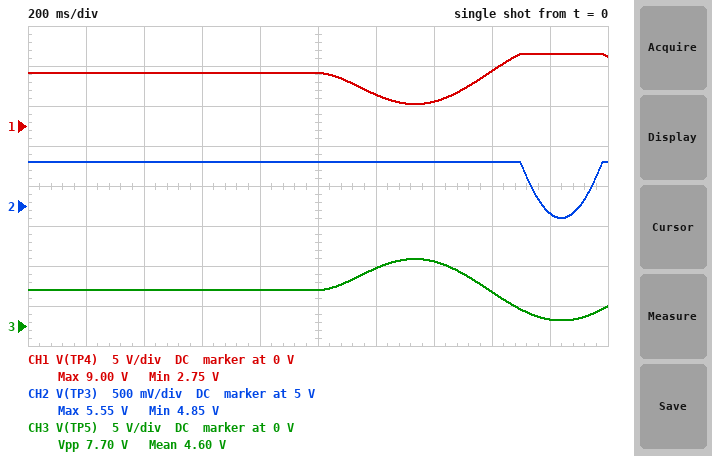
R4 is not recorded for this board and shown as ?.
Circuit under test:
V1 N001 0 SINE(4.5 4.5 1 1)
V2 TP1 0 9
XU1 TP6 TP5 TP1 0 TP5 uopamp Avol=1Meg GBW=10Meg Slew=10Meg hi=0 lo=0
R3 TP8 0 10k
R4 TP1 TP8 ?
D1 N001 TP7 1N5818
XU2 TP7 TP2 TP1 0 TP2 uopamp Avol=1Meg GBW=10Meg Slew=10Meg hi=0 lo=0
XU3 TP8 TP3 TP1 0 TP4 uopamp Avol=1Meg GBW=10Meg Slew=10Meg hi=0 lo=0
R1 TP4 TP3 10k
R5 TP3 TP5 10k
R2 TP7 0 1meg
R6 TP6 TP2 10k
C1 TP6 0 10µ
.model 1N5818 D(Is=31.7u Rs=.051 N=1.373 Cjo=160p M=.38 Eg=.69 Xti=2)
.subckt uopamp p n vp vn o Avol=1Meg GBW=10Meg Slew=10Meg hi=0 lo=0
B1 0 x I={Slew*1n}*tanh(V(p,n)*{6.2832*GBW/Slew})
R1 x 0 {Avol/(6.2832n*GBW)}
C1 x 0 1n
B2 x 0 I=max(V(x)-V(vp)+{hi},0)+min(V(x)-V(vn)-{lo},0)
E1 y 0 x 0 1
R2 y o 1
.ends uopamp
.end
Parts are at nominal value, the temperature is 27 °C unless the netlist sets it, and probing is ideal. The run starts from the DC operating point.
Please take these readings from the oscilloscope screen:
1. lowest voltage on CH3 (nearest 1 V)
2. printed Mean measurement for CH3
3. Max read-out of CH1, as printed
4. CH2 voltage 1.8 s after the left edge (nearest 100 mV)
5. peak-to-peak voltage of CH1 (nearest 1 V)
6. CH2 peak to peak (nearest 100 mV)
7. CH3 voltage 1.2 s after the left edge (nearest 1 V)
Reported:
1 V
4.60 V
9.00 V
4.9 V
6 V
700 mV
7 V
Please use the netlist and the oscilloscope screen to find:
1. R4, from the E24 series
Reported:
6.2 kΩ
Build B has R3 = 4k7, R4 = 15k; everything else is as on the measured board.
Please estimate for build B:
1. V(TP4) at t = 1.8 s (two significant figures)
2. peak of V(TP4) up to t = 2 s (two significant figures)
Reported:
3.5 V
3.6 V
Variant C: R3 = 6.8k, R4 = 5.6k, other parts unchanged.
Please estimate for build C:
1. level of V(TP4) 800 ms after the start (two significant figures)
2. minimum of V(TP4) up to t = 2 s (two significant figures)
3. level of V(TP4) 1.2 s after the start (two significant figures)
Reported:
5.4 V
1.5 V
2.7 V
